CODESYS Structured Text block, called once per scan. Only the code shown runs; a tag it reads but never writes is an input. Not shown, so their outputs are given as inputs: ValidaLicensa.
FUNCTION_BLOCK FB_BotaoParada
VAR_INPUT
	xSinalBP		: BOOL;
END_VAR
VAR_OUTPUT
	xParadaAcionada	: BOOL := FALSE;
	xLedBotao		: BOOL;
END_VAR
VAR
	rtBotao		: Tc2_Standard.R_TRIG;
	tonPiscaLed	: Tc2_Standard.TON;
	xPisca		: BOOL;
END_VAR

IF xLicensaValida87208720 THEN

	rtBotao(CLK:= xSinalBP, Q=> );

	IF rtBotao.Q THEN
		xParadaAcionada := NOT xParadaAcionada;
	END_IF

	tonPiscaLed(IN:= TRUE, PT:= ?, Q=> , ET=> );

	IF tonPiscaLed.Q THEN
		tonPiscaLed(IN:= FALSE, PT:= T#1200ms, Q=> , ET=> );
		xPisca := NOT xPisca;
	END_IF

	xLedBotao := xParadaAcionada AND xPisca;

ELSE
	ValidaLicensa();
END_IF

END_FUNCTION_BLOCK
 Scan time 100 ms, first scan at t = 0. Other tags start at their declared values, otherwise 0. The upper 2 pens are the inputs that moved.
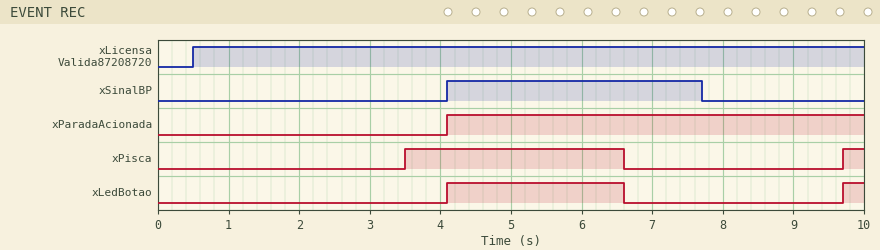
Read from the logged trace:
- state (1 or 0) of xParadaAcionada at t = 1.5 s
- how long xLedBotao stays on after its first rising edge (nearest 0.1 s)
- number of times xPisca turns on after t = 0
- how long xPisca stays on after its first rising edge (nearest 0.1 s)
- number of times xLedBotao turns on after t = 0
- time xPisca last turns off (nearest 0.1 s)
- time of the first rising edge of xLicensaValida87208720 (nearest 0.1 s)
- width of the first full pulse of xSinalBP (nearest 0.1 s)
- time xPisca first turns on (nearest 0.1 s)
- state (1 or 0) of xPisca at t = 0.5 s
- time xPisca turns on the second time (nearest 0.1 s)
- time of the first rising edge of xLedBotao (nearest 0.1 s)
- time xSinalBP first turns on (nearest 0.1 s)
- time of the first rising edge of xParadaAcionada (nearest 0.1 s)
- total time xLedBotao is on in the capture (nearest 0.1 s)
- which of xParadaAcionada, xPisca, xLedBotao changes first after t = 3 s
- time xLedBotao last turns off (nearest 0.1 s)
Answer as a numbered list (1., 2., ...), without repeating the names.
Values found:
1. 0
2. 2.5 s
3. 2
4. 3.1 s
5. 2
6. 6.6 s
7. 0.5 s
8. 3.6 s
9. 3.5 s
10. 0
11. 9.7 s
12. 4.1 s
13. 4.1 s
14. 4.1 s
15. 2.8 s
16. xPisca
17. 6.6 s
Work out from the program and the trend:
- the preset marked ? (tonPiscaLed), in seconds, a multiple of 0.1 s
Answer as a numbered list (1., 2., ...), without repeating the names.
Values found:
1. 3.0 s
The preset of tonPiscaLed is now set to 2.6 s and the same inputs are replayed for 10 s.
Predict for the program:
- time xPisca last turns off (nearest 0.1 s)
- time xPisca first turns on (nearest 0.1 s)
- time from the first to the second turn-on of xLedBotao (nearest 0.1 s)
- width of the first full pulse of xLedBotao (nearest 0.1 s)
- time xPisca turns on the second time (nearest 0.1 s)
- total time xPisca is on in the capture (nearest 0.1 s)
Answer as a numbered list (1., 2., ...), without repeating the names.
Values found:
1. 5.8 s
2. 3.1 s
3. 4.4 s
4. 1.7 s
5. 8.5 s
6. 4.2 s
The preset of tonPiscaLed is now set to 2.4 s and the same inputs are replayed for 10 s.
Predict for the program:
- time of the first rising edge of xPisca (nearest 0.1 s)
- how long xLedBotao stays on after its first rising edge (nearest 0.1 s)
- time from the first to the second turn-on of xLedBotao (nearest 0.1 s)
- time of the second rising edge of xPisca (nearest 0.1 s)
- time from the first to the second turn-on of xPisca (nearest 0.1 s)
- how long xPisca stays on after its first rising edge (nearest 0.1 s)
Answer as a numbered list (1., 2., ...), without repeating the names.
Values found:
1. 2.9 s
2. 1.3 s
3. 3.8 s
4. 7.9 s
5. 5.0 s
6. 2.5 s
